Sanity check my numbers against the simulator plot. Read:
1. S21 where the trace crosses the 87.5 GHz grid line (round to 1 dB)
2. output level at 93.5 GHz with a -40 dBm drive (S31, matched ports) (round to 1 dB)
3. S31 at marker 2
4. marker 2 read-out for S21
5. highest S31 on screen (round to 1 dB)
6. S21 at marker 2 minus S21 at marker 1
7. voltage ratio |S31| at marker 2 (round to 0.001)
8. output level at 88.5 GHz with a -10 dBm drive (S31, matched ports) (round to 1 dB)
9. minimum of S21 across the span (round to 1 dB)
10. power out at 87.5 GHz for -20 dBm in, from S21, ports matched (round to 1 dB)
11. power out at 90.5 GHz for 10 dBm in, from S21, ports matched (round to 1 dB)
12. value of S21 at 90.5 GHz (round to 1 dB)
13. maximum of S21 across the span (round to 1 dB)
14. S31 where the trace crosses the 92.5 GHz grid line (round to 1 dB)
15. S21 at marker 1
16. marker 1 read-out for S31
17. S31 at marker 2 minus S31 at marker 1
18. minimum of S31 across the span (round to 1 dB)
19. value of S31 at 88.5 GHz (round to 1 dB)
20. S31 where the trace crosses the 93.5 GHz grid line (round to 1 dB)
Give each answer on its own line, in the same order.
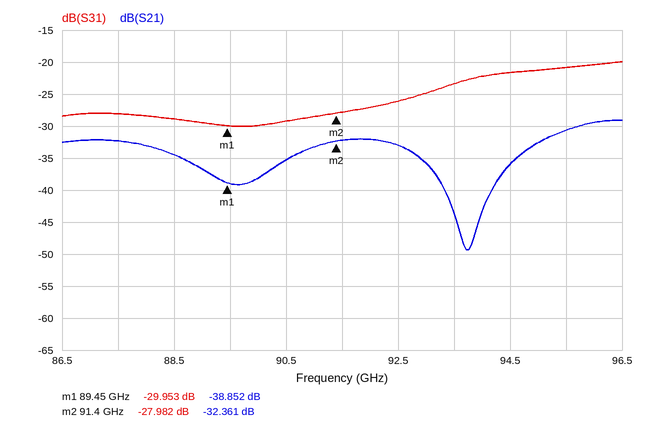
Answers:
-32 dB
-63 dBm
-27.982 dB
-32.361 dB
-20 dB
6.491 dB
0.040
-39 dBm
-49 dB
-52 dBm
-25 dBm
-35 dB
-29 dB
-26 dB
-38.852 dB
-29.953 dB
1.971 dB
-30 dB
-29 dB
-23 dB
